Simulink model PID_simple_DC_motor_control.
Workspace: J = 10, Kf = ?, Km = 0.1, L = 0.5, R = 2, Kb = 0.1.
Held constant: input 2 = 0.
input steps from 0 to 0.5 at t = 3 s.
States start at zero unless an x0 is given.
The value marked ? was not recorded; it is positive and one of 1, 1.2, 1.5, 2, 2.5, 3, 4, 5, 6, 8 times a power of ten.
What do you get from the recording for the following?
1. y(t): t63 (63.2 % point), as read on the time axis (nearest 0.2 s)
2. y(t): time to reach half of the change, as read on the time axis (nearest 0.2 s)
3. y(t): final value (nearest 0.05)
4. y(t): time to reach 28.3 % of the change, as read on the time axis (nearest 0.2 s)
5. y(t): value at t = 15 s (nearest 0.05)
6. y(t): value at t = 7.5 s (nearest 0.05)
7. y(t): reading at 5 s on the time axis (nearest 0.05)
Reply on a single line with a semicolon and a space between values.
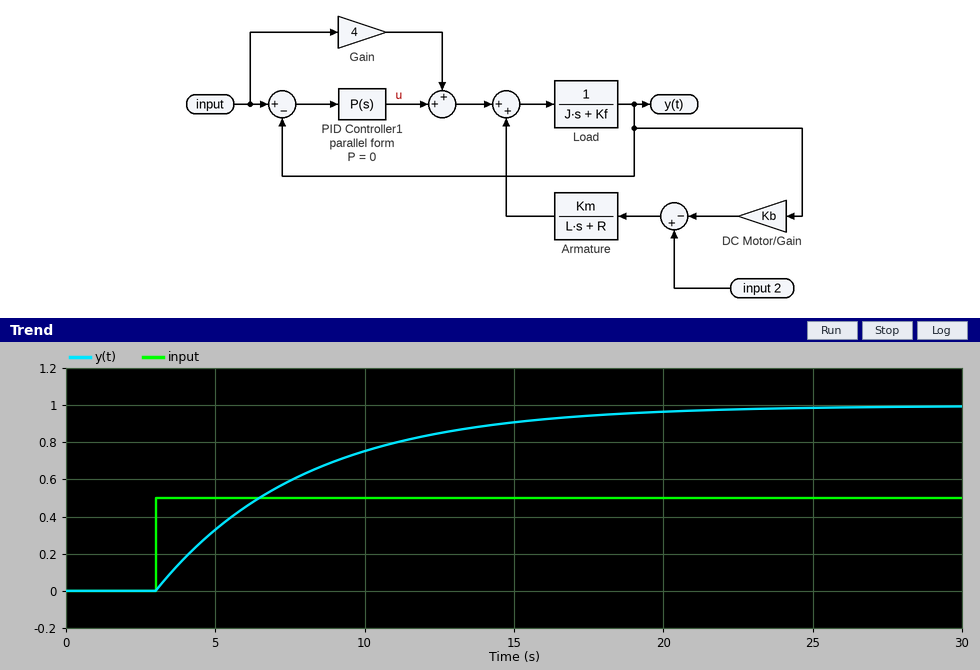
8.0 s; 6.4 s; 1.00; 4.6 s; 0.90; 0.60; 0.35
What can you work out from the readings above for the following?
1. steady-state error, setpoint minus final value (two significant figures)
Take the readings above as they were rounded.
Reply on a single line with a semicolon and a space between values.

-0.50
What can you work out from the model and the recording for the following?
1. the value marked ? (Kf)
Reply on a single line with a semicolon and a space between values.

2
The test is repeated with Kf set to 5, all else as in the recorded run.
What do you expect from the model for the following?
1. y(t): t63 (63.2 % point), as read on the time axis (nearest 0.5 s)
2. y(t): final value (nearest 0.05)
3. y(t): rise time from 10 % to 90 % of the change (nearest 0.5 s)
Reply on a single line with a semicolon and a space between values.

5.0 s; 0.40; 4.5 s
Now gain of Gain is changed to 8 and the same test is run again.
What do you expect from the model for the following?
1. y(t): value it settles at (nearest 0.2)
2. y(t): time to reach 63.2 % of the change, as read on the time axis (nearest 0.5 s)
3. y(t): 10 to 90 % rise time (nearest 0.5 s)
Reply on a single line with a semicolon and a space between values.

2.0; 8.0 s; 11.0 s
